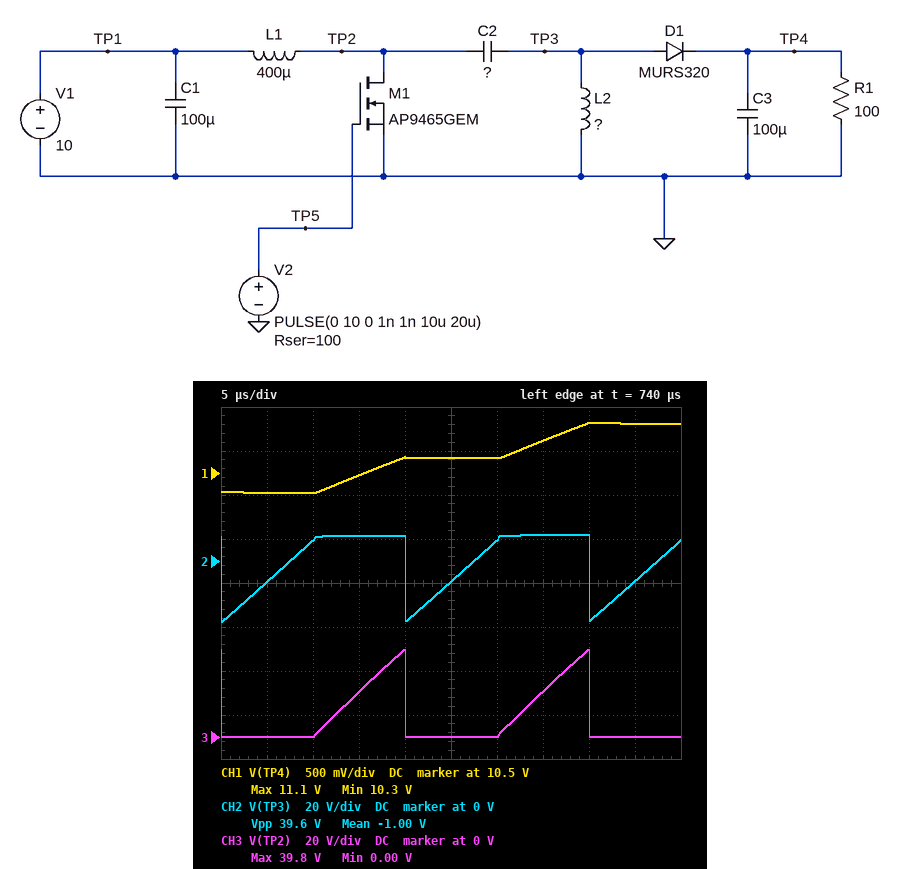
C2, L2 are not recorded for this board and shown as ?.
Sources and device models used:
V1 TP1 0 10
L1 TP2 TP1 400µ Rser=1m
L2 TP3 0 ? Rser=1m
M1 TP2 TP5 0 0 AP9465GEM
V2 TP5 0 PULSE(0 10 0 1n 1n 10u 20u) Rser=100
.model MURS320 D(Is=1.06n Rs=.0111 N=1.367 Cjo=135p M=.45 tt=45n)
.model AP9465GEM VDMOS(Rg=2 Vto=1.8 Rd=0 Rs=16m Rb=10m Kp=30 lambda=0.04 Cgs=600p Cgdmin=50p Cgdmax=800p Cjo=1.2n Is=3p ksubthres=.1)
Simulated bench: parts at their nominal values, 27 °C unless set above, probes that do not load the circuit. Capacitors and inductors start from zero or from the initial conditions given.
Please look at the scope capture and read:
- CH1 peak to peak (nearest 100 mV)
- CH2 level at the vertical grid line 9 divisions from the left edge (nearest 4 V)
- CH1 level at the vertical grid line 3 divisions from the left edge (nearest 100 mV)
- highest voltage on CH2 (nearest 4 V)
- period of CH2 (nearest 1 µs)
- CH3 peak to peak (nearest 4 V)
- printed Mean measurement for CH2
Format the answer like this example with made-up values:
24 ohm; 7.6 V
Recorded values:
800 mV; -8 V; 10.5 V; 12 V; 20 µs; 40 V; -1.00 V
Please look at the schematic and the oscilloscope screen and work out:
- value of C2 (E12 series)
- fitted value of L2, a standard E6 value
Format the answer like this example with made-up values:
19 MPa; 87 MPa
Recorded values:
560 nF; 1.5 mH
